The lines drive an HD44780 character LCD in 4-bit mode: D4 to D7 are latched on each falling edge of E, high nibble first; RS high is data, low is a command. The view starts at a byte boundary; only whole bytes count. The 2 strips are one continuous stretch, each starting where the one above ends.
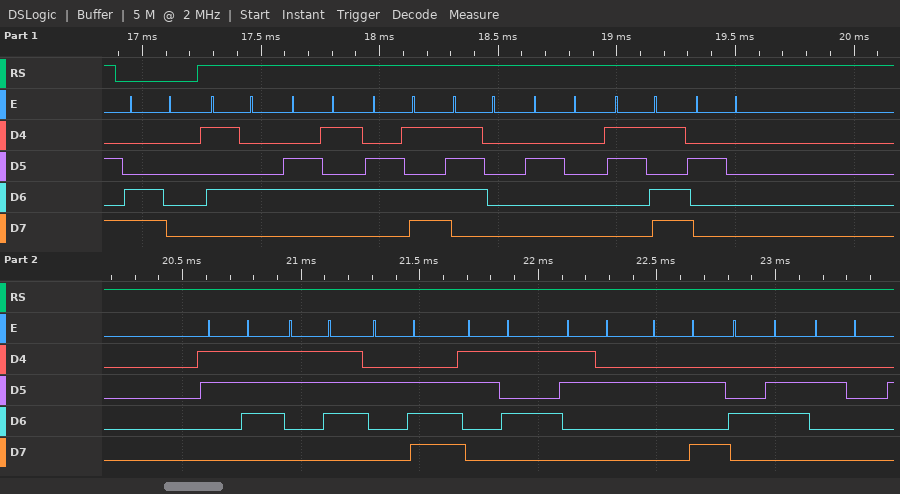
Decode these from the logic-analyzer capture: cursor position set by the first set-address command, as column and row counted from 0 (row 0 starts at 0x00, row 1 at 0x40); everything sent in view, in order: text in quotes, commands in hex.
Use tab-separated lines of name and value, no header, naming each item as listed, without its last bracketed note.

cursor position set by the first set-address command, as column and row counted from 0	column 0, row 1
everything sent in view, in order: text in quotes, commands in hex	0xC0 "Temp = 77.52*F "
